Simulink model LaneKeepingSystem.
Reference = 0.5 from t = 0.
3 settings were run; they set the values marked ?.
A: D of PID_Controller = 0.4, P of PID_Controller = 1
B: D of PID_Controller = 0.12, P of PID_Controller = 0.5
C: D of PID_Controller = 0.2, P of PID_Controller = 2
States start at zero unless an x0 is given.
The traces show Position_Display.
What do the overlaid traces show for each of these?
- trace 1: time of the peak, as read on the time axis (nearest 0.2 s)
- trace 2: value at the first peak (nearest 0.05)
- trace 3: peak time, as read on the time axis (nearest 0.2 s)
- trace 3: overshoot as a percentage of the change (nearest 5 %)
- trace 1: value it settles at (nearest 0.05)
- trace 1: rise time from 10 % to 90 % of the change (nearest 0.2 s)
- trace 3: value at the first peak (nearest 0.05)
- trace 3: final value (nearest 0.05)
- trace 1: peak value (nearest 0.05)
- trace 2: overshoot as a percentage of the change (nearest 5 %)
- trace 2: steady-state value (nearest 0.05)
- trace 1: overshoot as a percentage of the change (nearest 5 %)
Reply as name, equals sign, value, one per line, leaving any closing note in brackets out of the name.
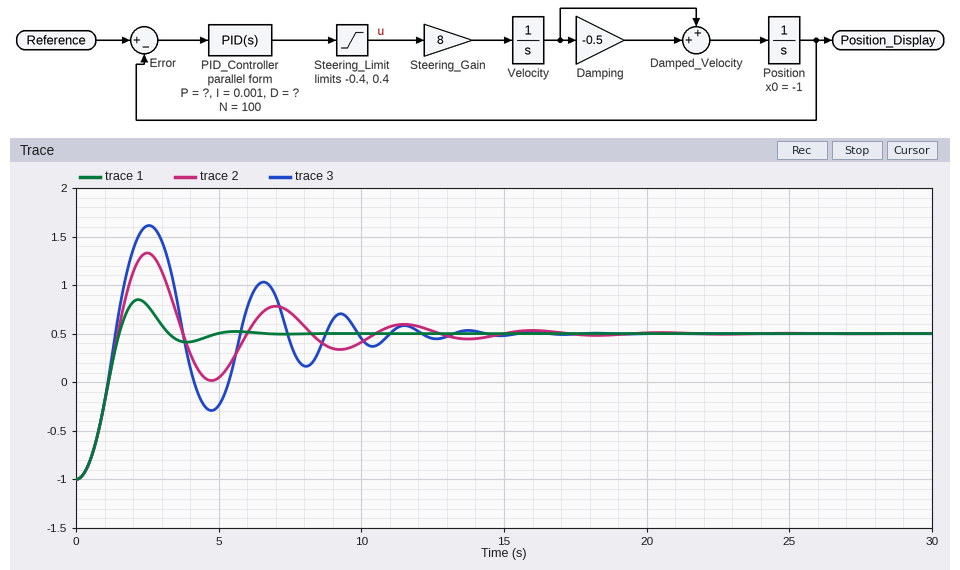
trace 1: time of the peak, as read on the time axis = 2.2 s
trace 2: value at the first peak = 1.35
trace 3: peak time, as read on the time axis = 2.6 s
trace 3: overshoot as a percentage of the change = 75 %
trace 1: value it settles at = 0.50
trace 1: rise time from 10 % to 90 % of the change = 1.0 s
trace 3: value at the first peak = 1.60
trace 3: final value = 0.50
trace 1: peak value = 0.85
trace 2: overshoot as a percentage of the change = 55 %
trace 2: steady-state value = 0.50
trace 1: overshoot as a percentage of the change = 25 %
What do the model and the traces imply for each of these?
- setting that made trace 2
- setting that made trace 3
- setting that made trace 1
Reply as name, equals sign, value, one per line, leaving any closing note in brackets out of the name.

setting that made trace 2 = B
setting that made trace 3 = C
setting that made trace 1 = A
